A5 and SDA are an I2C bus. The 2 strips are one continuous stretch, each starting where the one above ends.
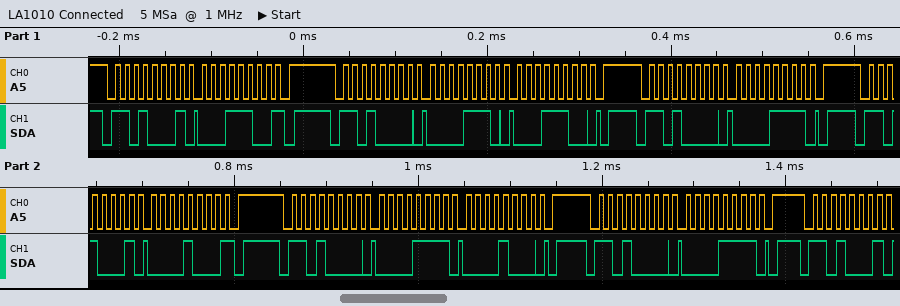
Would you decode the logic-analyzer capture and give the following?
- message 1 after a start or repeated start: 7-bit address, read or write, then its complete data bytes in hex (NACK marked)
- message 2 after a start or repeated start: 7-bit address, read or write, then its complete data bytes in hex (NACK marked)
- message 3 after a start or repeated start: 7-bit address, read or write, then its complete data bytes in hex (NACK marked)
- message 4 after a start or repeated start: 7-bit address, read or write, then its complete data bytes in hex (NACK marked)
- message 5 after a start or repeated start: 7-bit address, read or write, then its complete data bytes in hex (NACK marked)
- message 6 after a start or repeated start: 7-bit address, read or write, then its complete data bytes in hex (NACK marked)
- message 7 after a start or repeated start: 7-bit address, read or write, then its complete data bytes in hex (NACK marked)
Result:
0x68 read: 1C NACK
0x68 write: 0E 1C
0x68 write: 0F
0x68 read: 08 NACK
0x68 write: 0F 08
0x68 write: 0F
0x68 read
